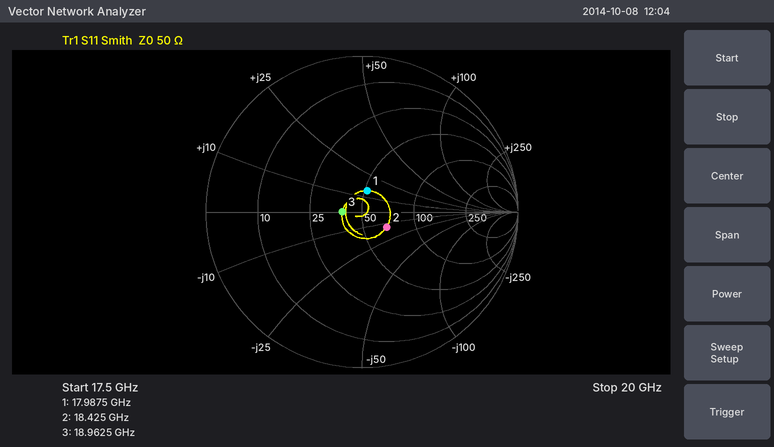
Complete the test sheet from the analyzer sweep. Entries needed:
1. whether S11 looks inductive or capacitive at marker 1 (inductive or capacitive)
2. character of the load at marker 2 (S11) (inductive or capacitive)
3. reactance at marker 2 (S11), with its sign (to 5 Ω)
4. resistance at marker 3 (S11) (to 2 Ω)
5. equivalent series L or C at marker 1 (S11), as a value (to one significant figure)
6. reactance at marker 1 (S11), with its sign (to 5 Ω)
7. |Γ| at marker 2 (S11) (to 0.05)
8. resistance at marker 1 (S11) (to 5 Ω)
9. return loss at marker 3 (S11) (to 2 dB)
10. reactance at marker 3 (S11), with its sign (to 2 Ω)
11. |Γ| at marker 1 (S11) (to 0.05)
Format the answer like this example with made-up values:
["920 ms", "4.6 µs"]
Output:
["inductive", "capacitive", "-15 Ω", "38 Ω", "100 pH", "+15 Ω", "0.20", "50 Ω", "18 dB", "0 Ω", "0.15"]
